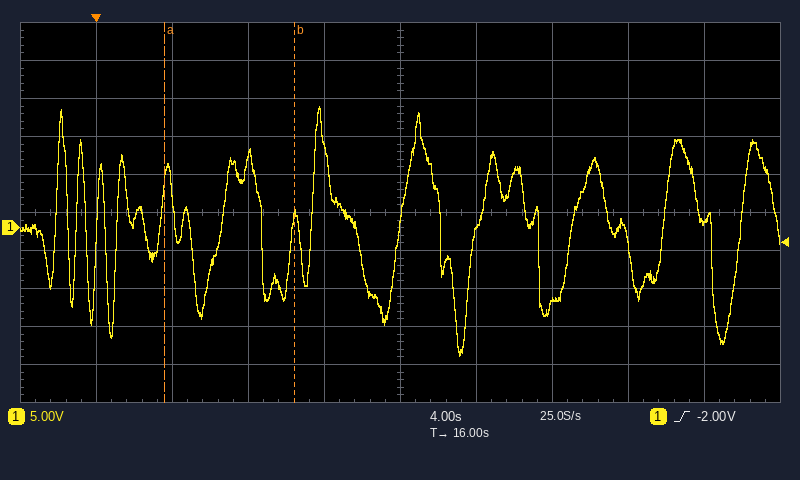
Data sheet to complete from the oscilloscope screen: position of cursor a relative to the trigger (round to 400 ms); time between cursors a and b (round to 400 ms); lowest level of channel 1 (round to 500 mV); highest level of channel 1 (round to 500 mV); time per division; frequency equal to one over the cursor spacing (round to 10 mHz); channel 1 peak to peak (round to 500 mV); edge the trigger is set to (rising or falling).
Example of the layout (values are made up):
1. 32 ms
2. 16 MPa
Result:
1. +3.6 s
2. 6.8 s
3. -17.0 V
4. 16.0 V
5. 4 s
6. 150 mHz
7. 33.0 V
8. rising
